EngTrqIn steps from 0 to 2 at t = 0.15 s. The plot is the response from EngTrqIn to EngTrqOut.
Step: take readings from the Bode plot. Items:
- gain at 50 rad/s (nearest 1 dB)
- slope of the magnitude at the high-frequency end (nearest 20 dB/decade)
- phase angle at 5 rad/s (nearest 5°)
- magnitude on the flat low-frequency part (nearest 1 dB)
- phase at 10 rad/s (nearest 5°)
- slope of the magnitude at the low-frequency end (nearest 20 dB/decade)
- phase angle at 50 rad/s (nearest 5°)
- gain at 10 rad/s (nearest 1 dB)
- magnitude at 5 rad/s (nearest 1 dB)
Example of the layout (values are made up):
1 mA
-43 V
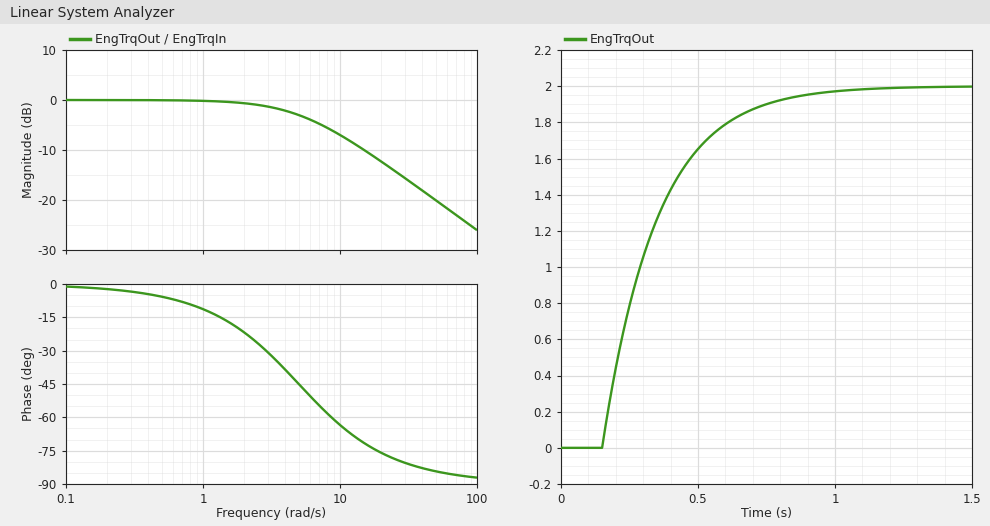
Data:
-20 dB
-20 dB/decade
-45°
0 dB
-65°
0 dB/decade
-85°
-7 dB
-3 dB
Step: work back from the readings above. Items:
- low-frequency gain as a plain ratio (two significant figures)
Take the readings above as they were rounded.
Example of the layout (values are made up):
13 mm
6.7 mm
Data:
1.0
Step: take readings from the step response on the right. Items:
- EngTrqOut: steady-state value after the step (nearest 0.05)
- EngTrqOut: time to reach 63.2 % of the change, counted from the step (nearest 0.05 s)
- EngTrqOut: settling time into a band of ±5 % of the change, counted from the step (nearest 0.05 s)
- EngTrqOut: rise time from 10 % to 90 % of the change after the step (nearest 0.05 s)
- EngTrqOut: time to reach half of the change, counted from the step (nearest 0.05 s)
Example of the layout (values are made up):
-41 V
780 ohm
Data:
2.00
0.20 s
0.60 s
0.45 s
0.15 s
